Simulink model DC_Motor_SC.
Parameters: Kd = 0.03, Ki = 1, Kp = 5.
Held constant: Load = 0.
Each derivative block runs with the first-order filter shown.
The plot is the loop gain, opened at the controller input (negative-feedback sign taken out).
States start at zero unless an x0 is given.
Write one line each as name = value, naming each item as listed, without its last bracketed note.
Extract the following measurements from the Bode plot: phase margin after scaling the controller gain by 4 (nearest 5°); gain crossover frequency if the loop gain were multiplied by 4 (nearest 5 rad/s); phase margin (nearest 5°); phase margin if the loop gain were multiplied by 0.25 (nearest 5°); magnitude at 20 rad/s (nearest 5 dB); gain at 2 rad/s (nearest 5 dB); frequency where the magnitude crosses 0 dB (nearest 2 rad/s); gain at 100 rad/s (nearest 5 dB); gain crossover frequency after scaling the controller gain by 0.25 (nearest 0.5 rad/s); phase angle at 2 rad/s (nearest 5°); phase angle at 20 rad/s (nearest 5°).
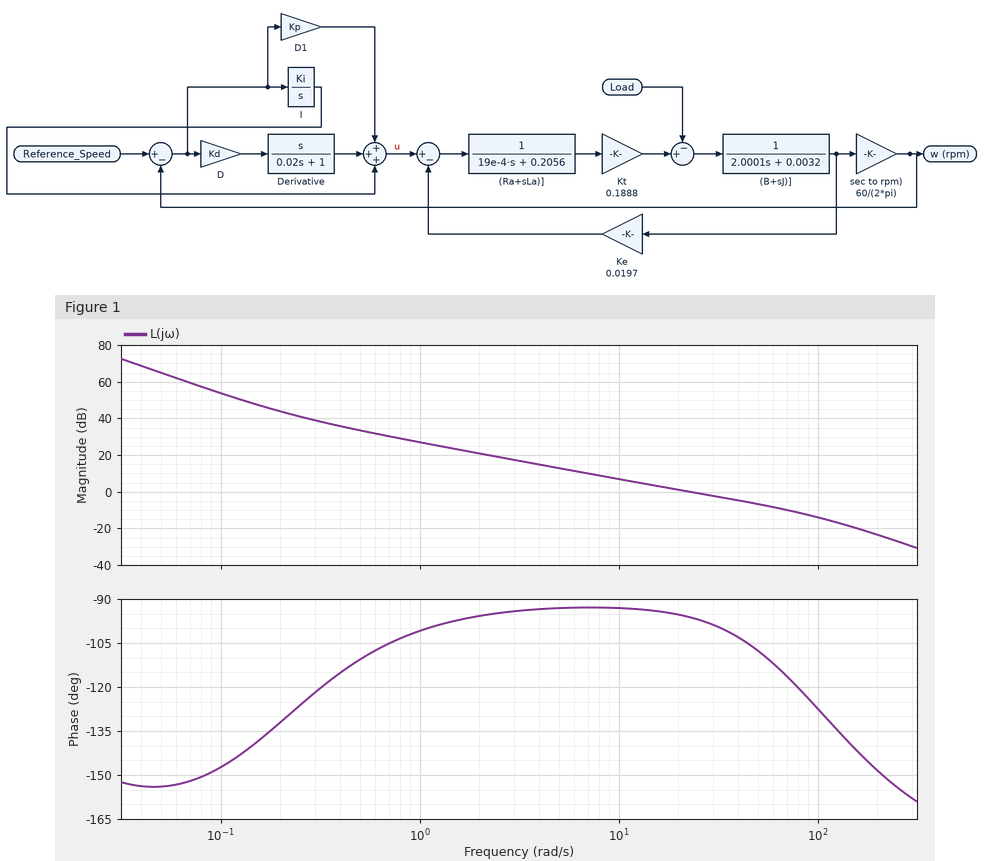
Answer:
phase margin after scaling the controller gain by 4 = 60°
gain crossover frequency if the loop gain were multiplied by 4 = 85 rad/s
phase margin = 85°
phase margin if the loop gain were multiplied by 0.25 = 85°
magnitude at 20 rad/s = 0 dB
gain at 2 rad/s = 20 dB
frequency where the magnitude crosses 0 dB = 22 rad/s
gain at 100 rad/s = -15 dB
gain crossover frequency after scaling the controller gain by 0.25 = 5.5 rad/s
phase angle at 2 rad/s = -95°
phase angle at 20 rad/s = -95°
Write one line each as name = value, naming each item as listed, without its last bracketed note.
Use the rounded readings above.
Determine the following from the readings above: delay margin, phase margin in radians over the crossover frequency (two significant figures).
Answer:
delay margin, phase margin in radians over the crossover frequency = 0.067 s
